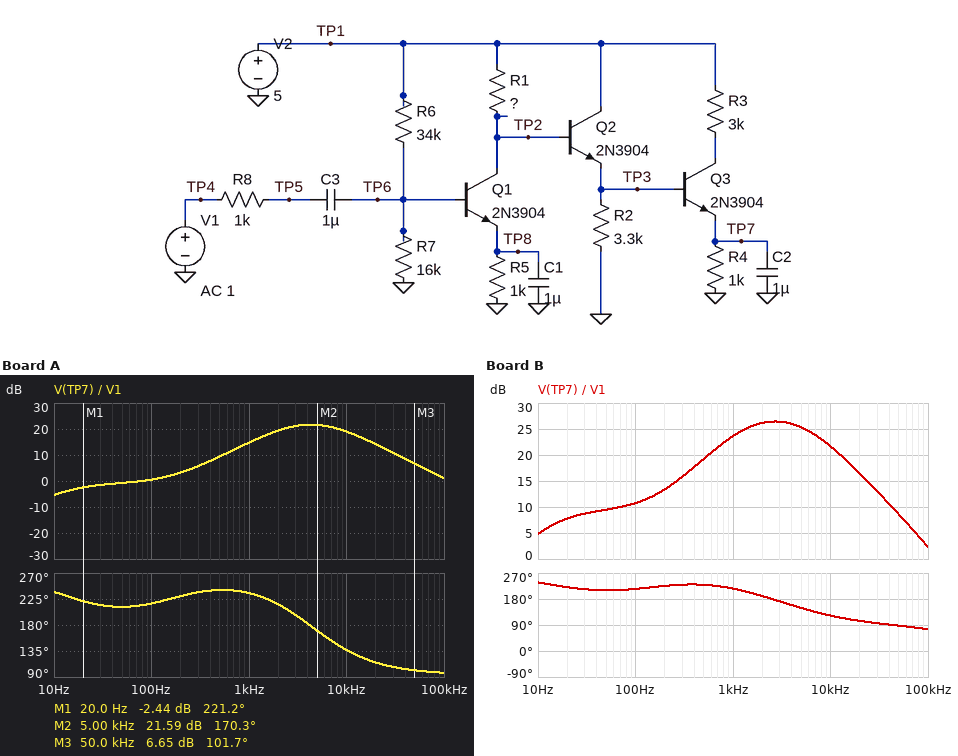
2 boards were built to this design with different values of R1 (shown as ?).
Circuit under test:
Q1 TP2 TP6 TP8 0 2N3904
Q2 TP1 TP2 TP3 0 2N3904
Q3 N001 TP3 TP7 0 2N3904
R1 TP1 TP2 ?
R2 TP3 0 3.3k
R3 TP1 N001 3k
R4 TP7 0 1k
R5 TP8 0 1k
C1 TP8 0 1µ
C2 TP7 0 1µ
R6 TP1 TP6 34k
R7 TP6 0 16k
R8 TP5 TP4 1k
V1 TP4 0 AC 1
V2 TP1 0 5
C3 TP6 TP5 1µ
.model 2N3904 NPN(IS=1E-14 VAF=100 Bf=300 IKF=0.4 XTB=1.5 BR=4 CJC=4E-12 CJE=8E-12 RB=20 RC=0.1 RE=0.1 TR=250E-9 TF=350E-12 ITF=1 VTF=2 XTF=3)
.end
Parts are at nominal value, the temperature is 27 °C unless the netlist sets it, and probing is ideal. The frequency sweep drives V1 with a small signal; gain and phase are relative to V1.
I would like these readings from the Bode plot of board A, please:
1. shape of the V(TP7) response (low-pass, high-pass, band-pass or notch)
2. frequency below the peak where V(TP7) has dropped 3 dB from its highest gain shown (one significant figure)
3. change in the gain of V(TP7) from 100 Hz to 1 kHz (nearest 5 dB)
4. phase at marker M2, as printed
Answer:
band-pass
2 kHz
15 dB
170.3 deg
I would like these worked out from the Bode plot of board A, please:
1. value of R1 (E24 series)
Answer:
1.1 kΩ
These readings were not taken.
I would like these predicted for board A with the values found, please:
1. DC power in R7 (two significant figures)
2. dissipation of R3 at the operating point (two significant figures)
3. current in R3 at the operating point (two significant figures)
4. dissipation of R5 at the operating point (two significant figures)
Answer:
150 µW
2.0 mW
810 µA
840 µW
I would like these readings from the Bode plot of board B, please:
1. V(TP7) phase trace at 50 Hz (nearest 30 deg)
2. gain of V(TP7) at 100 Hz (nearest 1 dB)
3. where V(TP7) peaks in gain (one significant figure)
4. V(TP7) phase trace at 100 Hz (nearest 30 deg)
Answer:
210 deg
11 dB
3 kHz
210 deg
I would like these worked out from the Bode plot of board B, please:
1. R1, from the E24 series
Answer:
3.9 kΩ
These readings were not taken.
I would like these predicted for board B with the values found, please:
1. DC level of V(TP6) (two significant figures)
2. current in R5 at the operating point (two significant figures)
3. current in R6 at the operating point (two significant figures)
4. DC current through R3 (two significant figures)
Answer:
1.6 V
910 µA
100 µA
210 µA
